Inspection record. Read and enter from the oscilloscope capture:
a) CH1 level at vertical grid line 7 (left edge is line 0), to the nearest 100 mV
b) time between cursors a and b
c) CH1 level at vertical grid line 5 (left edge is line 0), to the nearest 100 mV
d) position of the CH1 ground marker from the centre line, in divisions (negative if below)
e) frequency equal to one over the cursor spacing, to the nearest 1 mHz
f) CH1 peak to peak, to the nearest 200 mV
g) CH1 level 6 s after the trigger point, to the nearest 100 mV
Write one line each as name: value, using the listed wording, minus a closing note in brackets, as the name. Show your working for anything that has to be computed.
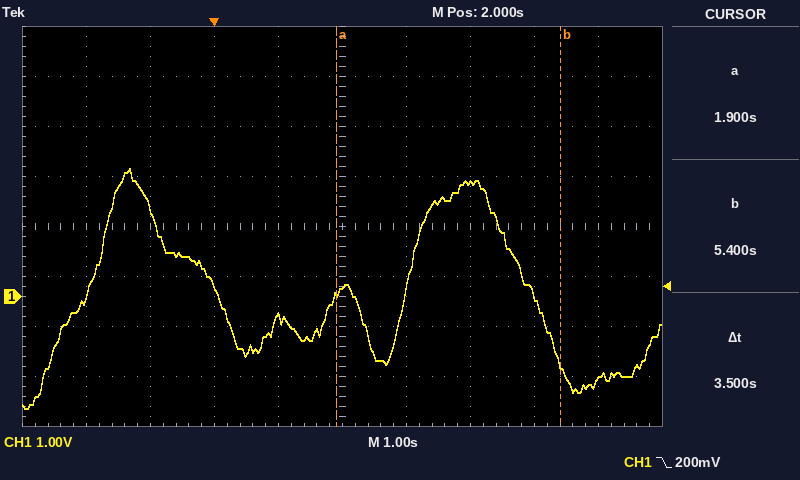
CH1 level at vertical grid line 7 (left edge is line 0), to the nearest 100 mV: 2.3 V
time between cursors a and b: 3.5 s
CH1 level at vertical grid line 5 (left edge is line 0), to the nearest 100 mV: 200 mV
position of the CH1 ground marker from the centre line, in divisions: -1.4 div
frequency equal to one over the cursor spacing, to the nearest 1 mHz: 1 / 3.5 s ≈ 286 mHz
CH1 peak to peak, to the nearest 200 mV: 4.8 V
CH1 level 6 s after the trigger point, to the nearest 100 mV: -1.7 V
